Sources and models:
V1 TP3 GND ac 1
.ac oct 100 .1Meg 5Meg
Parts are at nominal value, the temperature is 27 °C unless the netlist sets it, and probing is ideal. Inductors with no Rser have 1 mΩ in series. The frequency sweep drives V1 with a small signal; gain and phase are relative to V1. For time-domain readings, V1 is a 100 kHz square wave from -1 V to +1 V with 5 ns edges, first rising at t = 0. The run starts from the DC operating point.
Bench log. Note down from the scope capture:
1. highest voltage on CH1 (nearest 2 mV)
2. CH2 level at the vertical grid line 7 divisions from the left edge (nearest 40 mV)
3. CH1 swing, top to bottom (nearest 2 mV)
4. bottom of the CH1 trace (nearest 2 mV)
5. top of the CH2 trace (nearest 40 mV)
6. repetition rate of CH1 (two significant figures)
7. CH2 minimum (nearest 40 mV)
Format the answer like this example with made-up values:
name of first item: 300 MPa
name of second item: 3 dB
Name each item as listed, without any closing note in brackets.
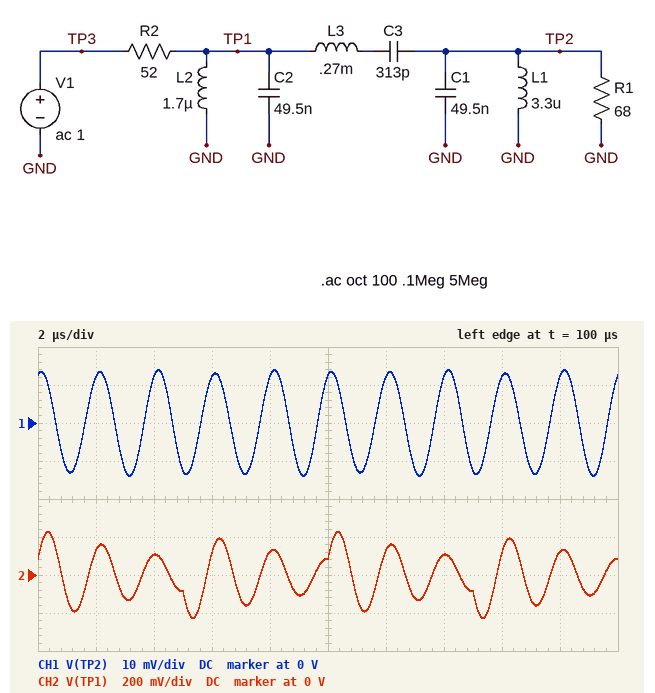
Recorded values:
highest voltage on CH1: 14 mV
CH2 level at the vertical grid line 7 divisions from the left edge: 120 mV
CH1 swing, top to bottom: 28 mV
bottom of the CH1 trace: -14 mV
top of the CH2 trace: 240 mV
repetition rate of CH1: 500 kHz
CH2 minimum: -240 mV
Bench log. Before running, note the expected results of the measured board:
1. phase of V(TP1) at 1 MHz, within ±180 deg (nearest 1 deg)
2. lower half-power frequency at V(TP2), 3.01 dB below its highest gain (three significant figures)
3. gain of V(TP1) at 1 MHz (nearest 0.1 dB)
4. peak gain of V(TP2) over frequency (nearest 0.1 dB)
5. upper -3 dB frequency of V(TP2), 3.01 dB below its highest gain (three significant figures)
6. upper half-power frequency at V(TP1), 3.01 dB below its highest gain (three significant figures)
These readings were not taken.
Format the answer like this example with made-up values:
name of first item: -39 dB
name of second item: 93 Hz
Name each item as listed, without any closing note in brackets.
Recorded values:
phase of V(TP1) at 1 MHz, within ±180 deg: -85 deg
lower half-power frequency at V(TP2), 3.01 dB below its highest gain: 527 kHz
gain of V(TP1) at 1 MHz: -21.1 dB
peak gain of V(TP2) over frequency: -13.2 dB
upper -3 dB frequency of V(TP2), 3.01 dB below its highest gain: 571 kHz
upper half-power frequency at V(TP1), 3.01 dB below its highest gain: 594 kHz
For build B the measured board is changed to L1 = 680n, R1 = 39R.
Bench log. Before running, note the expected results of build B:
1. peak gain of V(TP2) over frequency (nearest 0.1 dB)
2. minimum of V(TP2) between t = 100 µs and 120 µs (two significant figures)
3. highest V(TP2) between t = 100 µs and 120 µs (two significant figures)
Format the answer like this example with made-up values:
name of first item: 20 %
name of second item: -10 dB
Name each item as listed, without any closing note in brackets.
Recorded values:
peak gain of V(TP2) over frequency: -22.7 dB
minimum of V(TP2) between t = 100 µs and 120 µs: -3.8 mV
highest V(TP2) between t = 100 µs and 120 µs: 3.8 mV
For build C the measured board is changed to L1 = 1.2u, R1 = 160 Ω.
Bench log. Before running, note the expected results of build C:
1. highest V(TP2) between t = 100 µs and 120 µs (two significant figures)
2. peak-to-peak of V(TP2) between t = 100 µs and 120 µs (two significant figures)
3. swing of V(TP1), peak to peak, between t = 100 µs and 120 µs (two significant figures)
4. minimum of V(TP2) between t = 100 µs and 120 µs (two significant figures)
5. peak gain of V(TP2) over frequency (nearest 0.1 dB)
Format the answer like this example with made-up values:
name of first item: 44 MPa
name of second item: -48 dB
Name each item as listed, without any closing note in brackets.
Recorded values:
highest V(TP2) between t = 100 µs and 120 µs: 12 mV
peak-to-peak of V(TP2) between t = 100 µs and 120 µs: 24 mV
swing of V(TP1), peak to peak, between t = 100 µs and 120 µs: 460 mV
minimum of V(TP2) between t = 100 µs and 120 µs: -12 mV
peak gain of V(TP2) over frequency: -12.0 dB
